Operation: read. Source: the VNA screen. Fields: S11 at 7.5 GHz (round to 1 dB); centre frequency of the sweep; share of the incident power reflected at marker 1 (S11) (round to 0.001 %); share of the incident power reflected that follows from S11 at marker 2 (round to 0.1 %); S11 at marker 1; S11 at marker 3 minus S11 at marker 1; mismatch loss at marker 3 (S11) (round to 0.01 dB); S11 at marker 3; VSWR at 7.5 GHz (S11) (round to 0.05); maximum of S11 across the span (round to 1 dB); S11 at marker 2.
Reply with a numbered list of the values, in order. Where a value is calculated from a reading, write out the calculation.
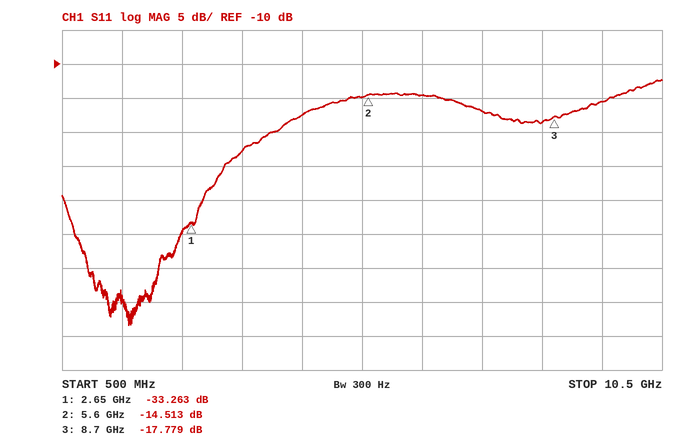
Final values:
1. -17 dB
2. 5.5 GHz
3. 10^(-33.263/10) ≈ 0.047 %
4. 10^(-14.513/10) ≈ 3.5 %
5. -33.263 dB
6. -17.779 − (-33.263) = 15.484 dB
7. −10 log10(1 − 10^(-17.779/10)) ≈ 0.07 dB
8. -17.779 dB
9. |Γ| = 10^(-17/20) = 0.1413; VSWR = (1 + 0.1413)/(1 − 0.1413) ≈ 1.33, so 1.35 to the nearest 0.05
10. -12 dB
11. -14.513 dB
